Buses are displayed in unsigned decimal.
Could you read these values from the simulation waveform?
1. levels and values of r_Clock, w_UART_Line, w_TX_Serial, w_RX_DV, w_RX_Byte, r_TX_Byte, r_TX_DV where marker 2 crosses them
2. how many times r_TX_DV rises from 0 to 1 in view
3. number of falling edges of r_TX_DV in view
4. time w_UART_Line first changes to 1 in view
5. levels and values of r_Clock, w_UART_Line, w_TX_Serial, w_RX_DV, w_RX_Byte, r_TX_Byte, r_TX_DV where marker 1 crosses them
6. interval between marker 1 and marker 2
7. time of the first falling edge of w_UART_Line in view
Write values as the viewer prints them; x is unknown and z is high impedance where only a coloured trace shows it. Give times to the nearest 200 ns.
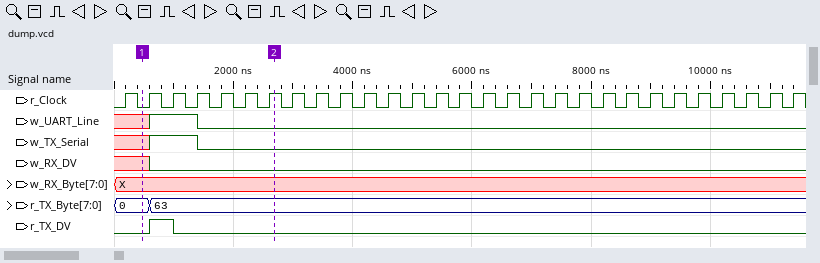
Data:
r_Clock=1, w_UART_Line=0, w_TX_Serial=0, w_RX_DV=0, w_RX_Byte=X, r_TX_Byte=63, r_TX_DV=0
1
1
600 ns
r_Clock=0, w_UART_Line=x, w_TX_Serial=x, w_RX_DV=x, w_RX_Byte=X, r_TX_Byte=0, r_TX_DV=0
2200 ns
1400 ns
